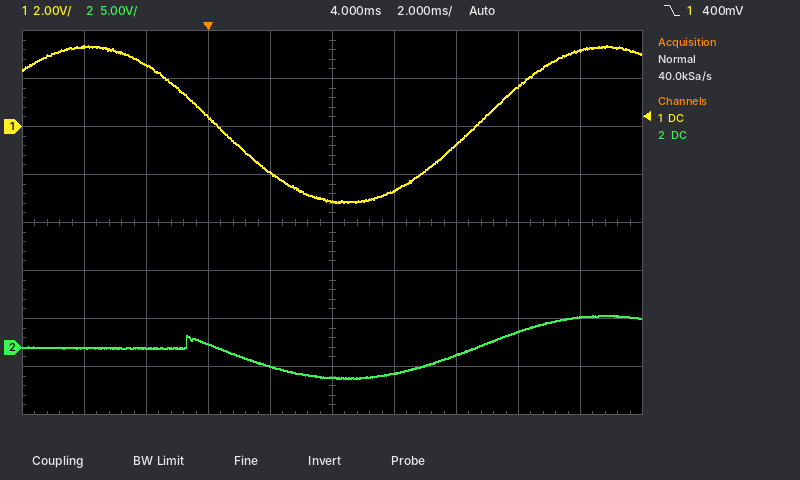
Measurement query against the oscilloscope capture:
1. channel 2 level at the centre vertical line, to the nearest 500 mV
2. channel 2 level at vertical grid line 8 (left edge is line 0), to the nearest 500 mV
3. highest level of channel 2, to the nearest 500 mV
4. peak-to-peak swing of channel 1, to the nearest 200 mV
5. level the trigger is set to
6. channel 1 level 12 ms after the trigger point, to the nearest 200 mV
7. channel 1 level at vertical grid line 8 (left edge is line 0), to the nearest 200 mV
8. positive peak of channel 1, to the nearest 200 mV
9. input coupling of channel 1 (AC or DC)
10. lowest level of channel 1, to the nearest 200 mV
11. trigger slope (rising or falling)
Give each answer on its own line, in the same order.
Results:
-3.0 V
1.5 V
3.5 V
6.6 V
400 mV
3.2 V
1.6 V
3.4 V
DC
-3.2 V
falling
